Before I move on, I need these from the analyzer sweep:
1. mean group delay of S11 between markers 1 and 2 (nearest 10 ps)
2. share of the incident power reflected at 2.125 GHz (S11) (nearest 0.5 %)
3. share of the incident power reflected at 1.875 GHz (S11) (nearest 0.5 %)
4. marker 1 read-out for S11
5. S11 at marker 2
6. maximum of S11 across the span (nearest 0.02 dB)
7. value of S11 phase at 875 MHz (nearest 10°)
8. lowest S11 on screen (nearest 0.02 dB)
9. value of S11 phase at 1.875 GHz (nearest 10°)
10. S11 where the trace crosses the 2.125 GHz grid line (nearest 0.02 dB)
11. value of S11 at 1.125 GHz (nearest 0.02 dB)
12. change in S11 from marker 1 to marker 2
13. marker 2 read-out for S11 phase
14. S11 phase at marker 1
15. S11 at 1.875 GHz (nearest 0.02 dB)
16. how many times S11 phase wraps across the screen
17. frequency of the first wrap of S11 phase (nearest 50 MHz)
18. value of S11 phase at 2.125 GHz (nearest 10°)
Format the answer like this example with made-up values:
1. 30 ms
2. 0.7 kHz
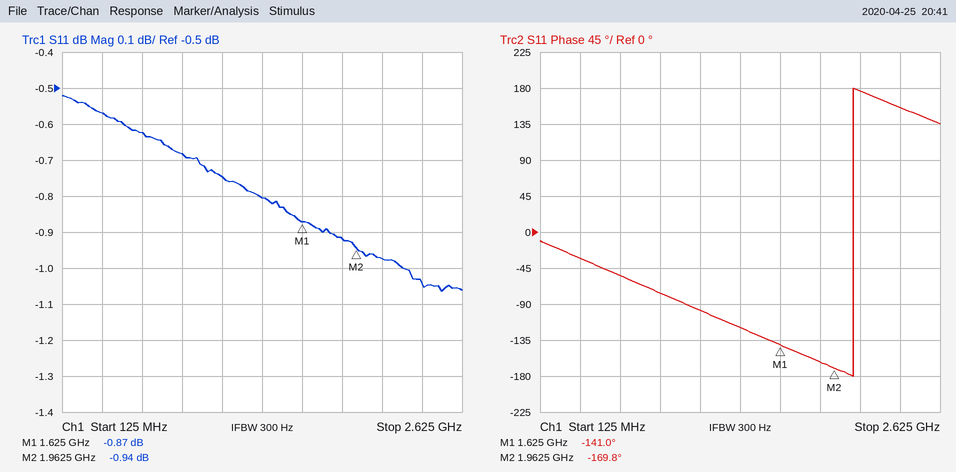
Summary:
1. 240 ps
2. 80.0 %
3. 81.0 %
4. -0.87 dB
5. -0.94 dB
6. -0.52 dB
7. -80°
8. -1.06 dB
9. -160°
10. -0.98 dB
11. -0.74 dB
12. -0.07 dB
13. -169.8°
14. -141.0°
15. -0.92 dB
16. 1
17. 2.10 GHz
18. 180°
